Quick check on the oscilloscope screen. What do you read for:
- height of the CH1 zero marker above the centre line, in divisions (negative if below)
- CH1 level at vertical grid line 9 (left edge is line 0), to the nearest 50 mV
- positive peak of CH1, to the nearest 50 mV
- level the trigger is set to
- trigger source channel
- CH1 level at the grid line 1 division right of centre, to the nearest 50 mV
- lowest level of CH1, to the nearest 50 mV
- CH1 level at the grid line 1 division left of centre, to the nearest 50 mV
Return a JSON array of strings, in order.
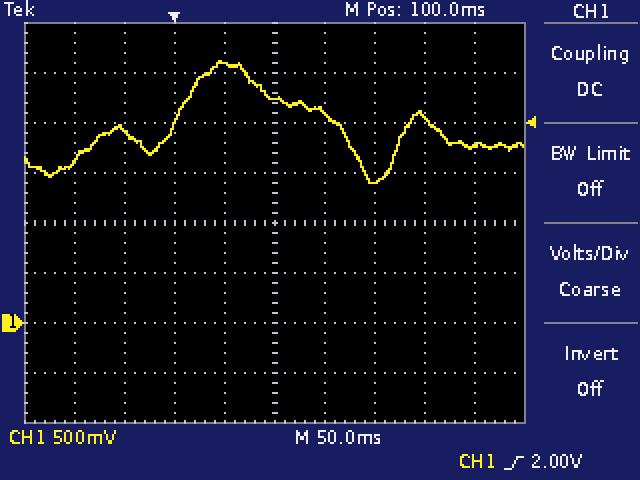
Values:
["-2.0 div", "1.75 V", "2.60 V", "2.00 V", "CH1", "2.10 V", "1.40 V", "2.60 V"]
